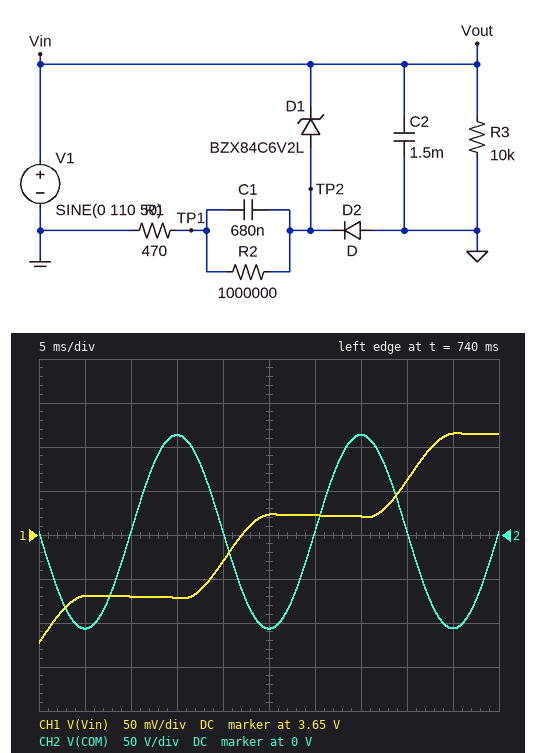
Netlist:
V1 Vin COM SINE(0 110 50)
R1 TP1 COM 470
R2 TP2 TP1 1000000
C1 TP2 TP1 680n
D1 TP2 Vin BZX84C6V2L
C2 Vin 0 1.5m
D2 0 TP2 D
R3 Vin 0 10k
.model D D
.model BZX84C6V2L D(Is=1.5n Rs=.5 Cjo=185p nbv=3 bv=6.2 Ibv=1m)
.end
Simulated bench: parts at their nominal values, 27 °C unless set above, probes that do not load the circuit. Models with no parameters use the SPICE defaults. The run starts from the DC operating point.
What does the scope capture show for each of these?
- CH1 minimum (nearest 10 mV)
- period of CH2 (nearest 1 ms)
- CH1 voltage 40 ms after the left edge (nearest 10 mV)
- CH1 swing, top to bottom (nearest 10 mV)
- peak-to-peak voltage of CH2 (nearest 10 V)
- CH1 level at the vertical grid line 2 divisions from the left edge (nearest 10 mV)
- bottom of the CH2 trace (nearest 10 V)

3.53 V
20 ms
3.71 V
240 mV
220 V
3.58 V
-110 V
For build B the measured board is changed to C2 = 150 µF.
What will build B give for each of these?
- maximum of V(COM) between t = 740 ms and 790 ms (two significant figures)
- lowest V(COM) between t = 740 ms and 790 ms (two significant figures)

120 V
-100 V
